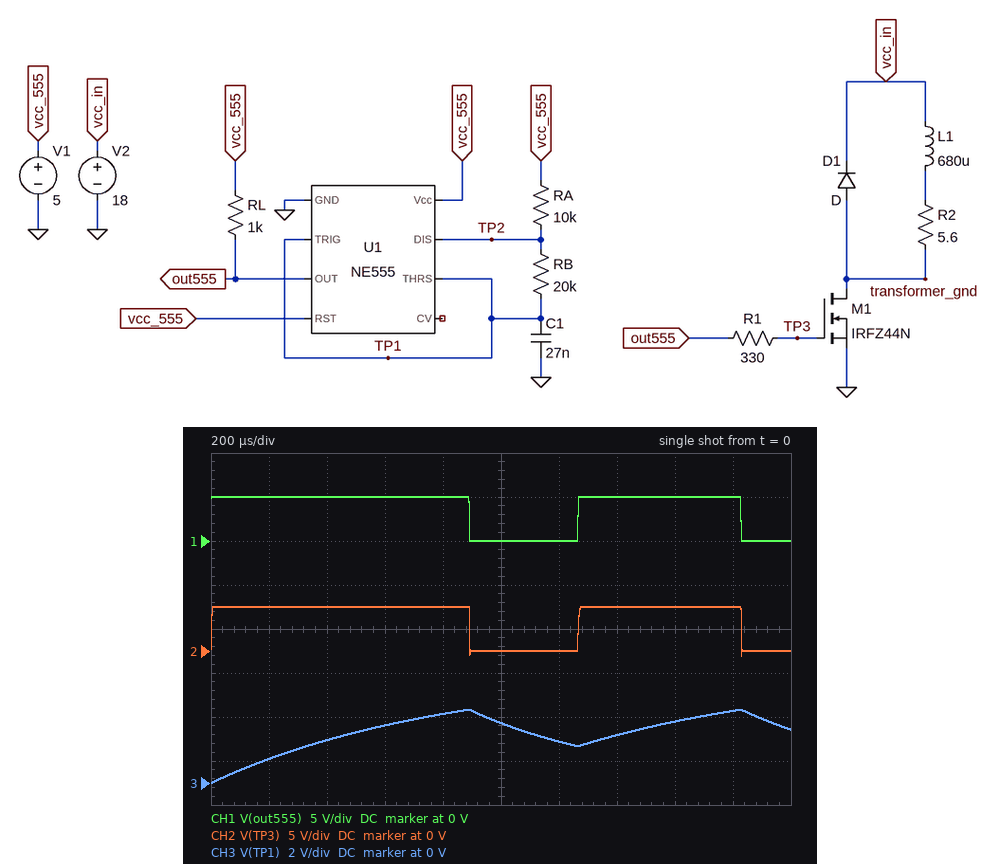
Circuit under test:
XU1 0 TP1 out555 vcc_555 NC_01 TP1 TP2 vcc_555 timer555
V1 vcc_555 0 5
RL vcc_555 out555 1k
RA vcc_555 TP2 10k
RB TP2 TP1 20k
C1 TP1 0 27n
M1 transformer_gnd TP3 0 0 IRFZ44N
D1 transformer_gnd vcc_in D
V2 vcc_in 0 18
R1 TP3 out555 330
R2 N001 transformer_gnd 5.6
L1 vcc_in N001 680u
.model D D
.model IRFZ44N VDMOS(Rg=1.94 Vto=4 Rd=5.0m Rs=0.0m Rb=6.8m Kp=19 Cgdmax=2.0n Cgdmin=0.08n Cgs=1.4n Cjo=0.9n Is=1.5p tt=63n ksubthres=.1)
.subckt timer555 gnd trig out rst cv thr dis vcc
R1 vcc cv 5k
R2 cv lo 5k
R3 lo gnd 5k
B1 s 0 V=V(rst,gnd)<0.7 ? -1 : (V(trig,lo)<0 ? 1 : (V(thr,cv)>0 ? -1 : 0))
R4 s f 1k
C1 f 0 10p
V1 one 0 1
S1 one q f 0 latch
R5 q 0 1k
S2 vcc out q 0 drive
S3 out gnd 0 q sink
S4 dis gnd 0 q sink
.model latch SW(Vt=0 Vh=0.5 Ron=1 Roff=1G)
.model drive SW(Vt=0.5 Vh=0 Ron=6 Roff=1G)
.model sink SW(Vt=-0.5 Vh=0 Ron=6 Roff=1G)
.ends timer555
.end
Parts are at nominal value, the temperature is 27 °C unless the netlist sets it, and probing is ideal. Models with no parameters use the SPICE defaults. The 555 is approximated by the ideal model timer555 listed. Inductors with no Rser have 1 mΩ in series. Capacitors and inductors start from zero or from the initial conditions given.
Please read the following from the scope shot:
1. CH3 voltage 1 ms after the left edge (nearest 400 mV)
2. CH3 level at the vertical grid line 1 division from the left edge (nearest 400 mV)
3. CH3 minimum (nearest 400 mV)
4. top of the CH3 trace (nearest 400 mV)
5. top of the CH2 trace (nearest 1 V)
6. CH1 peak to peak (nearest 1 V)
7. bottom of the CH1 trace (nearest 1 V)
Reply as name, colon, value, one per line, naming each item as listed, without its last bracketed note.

CH3 voltage 1 ms after the left edge: 2.8 V
CH3 level at the vertical grid line 1 division from the left edge: 1.2 V
CH3 minimum: 0 V
top of the CH3 trace: 3.2 V
top of the CH2 trace: 5 V
CH1 peak to peak: 5 V
bottom of the CH1 trace: 0 V
